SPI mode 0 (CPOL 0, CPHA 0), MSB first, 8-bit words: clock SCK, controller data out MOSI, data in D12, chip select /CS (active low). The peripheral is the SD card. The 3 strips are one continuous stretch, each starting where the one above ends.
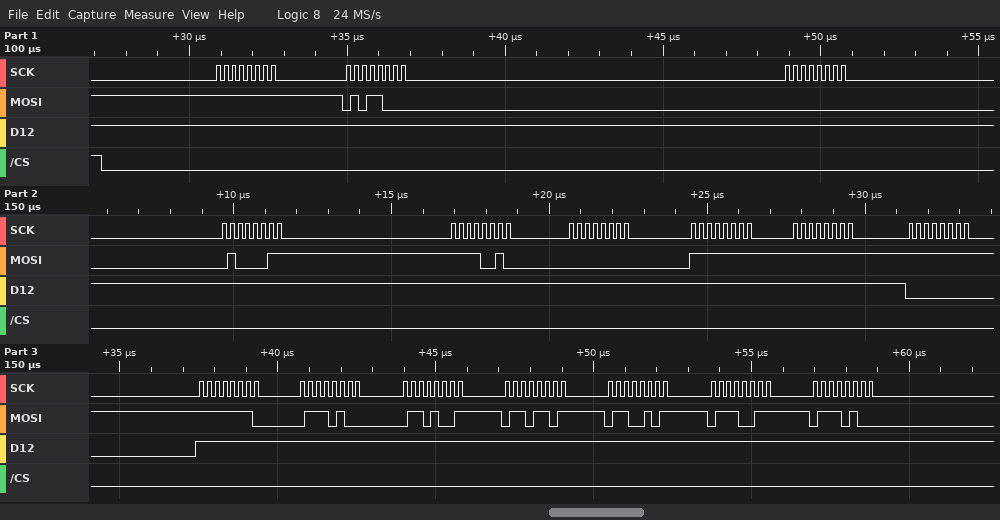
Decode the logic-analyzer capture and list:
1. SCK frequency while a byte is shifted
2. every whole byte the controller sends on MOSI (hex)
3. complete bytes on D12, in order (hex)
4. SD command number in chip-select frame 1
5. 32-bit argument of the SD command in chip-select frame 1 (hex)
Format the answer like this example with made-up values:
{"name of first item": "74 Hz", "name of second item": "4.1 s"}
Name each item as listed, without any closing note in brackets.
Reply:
{"SCK frequency while a byte is shifted": "4 MHz", "every whole byte the controller sends on MOSI": "FF 58 00 43 F2 00 FF FF FF FE 74 69 6D 65 73 74", "complete bytes on D12, in order": "FF FF FF FF FF FF FF FF 00 FF FF FF FF FF FF FF", "SD command number in chip-select frame 1": "CMD24", "32-bit argument of the SD command in chip-select frame 1": "0x0043F200"}
